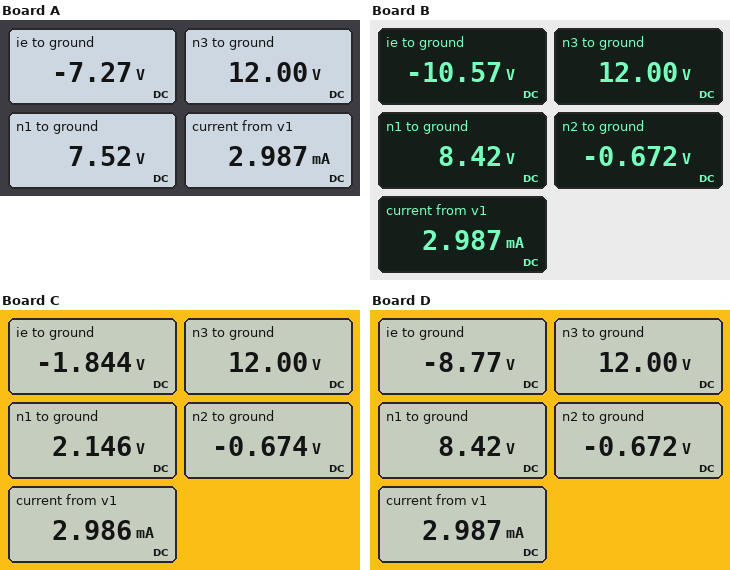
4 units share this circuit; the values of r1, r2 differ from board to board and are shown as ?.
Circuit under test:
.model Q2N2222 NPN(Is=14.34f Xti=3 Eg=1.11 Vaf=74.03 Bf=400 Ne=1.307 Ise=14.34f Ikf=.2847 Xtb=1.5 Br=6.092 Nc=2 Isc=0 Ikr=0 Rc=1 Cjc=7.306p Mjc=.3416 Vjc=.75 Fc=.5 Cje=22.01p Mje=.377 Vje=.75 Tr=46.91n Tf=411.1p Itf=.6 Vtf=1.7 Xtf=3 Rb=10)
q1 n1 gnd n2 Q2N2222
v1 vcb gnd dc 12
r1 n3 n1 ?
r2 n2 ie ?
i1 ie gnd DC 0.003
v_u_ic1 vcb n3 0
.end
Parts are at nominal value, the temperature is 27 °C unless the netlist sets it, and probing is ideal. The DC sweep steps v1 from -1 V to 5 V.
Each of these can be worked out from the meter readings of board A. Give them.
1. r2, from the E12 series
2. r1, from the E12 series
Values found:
2.2 kΩ
1.5 kΩ
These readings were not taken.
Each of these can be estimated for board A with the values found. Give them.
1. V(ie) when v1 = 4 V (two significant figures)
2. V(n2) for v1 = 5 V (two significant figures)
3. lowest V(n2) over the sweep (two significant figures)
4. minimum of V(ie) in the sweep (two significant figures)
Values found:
-7.3 V
-670 mV
-760 mV
-7.4 V
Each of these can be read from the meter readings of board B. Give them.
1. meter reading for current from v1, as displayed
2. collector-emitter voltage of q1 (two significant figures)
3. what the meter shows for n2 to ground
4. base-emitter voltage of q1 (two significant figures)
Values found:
2.987 mA
9.1 V
-0.672 V
670 mV
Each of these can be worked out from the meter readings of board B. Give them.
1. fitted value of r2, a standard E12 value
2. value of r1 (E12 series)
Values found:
3.3 kΩ
1.2 kΩ
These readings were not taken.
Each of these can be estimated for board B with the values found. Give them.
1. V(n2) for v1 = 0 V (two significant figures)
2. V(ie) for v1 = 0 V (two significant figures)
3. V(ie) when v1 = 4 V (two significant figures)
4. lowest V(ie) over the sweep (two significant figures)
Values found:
-740 mV
-11 V
-11 V
-11 V
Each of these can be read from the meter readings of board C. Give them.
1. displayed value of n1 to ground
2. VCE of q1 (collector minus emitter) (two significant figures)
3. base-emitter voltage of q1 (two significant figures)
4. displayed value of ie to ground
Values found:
2.146 V
2.8 V
670 mV
-1.844 V
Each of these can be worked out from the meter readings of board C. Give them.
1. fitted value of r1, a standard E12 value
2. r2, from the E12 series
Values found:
3.3 kΩ
390 Ω
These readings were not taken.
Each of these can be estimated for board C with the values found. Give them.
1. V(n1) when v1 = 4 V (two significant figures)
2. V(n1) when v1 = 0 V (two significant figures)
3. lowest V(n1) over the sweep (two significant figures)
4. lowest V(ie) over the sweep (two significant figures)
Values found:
-720 mV
-750 mV
-750 mV
-1.9 V
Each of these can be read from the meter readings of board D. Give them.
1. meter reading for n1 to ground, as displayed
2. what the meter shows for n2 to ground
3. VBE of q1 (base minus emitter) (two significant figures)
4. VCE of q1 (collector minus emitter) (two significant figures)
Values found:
8.42 V
-0.672 V
670 mV
9.1 V
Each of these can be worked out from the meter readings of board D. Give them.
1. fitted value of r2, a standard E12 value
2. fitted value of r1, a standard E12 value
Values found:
2.7 kΩ
1.2 kΩ
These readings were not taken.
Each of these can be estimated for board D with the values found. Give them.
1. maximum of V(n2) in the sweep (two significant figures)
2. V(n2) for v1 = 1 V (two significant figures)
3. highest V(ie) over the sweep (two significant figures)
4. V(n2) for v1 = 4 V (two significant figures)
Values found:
-670 mV
-730 mV
-8.8 V
-670 mV
